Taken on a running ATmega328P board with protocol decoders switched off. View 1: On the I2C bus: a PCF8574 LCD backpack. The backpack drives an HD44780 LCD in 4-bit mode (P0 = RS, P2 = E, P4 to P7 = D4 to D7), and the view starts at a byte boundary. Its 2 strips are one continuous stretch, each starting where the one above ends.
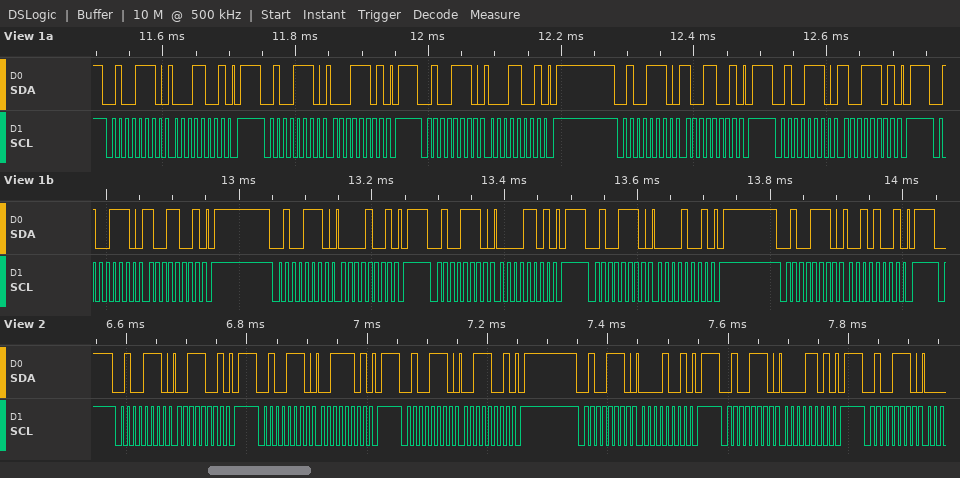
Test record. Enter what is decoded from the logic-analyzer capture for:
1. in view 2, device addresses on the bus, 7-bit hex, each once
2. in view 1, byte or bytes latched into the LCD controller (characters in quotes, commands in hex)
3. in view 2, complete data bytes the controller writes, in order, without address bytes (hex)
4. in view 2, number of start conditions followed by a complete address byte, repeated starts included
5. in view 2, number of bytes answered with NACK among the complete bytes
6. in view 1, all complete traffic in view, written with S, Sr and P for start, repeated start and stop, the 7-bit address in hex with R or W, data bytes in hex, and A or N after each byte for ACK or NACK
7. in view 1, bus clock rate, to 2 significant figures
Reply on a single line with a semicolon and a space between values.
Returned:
0x27; data 0x19; 39 3D 39 09 0D; 6; 0; S 27W A 19 A P S 27W A 1D A P S 27W A 19 A P S 27W A 99 A P S 27W A 9D A P S 27W A 99 A P S 27W A 09 A P S 27W A 0D A P S 27W A 09 A P S 27W A 29 A P; 100 kHz
